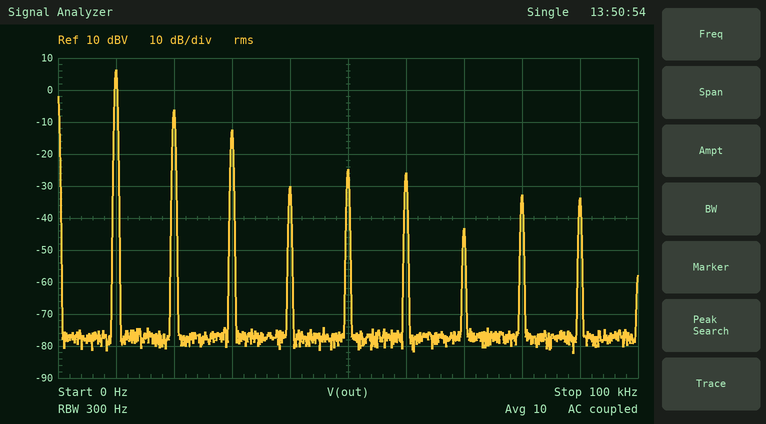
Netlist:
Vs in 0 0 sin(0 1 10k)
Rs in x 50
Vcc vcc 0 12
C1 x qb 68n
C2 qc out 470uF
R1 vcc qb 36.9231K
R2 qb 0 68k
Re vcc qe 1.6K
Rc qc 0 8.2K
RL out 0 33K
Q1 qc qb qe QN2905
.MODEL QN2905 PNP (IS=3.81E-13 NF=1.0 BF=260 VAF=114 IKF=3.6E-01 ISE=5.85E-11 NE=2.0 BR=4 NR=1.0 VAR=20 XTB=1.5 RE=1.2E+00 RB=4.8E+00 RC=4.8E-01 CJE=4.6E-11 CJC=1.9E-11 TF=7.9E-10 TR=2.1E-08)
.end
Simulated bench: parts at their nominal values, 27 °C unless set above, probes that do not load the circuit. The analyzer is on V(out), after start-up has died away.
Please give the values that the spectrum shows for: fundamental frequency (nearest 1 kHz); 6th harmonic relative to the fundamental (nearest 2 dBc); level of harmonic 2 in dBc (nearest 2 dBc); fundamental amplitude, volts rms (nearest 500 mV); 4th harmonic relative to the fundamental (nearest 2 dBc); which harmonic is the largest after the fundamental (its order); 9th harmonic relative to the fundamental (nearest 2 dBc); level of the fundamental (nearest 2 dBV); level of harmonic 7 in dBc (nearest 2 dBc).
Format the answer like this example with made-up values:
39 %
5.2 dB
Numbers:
10 kHz
-32 dBc
-12 dBc
2.0 V
-36 dBc
2
-40 dBc
6 dBV
-50 dBc
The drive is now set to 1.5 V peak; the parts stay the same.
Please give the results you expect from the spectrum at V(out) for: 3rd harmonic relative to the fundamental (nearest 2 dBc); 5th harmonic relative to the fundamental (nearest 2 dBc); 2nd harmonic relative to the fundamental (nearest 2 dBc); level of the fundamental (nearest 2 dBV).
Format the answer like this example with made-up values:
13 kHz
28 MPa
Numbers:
-16 dBc
-52 dBc
-16 dBc
10 dBV
